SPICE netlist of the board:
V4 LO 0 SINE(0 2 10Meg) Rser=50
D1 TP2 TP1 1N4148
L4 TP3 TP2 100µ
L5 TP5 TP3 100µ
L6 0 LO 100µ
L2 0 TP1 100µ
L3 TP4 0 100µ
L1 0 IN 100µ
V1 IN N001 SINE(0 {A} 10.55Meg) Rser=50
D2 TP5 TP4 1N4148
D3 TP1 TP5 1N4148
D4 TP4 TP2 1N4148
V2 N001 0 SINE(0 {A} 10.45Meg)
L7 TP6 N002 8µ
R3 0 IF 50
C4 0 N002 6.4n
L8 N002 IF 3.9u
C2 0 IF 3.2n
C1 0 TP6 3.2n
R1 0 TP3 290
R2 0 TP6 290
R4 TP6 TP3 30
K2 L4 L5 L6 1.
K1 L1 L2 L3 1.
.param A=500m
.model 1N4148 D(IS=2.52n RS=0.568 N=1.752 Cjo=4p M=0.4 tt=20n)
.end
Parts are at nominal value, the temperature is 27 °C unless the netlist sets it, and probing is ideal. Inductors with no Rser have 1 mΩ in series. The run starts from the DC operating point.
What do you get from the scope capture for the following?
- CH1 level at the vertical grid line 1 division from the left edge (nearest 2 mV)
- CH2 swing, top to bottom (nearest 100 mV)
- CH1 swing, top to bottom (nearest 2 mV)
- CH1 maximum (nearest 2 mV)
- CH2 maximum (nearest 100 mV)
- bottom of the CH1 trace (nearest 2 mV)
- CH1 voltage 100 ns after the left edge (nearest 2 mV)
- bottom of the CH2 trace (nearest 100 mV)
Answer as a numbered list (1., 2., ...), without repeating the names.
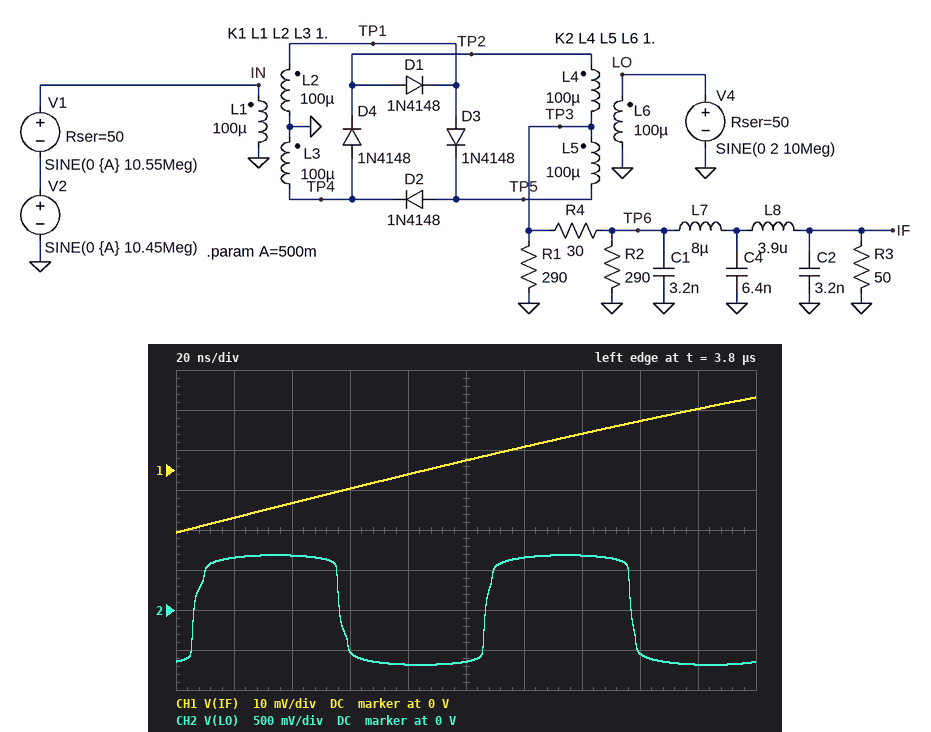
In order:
1. -12 mV
2. 1.4 V
3. 34 mV
4. 18 mV
5. 700 mV
6. -16 mV
7. 2 mV
8. -700 mV
